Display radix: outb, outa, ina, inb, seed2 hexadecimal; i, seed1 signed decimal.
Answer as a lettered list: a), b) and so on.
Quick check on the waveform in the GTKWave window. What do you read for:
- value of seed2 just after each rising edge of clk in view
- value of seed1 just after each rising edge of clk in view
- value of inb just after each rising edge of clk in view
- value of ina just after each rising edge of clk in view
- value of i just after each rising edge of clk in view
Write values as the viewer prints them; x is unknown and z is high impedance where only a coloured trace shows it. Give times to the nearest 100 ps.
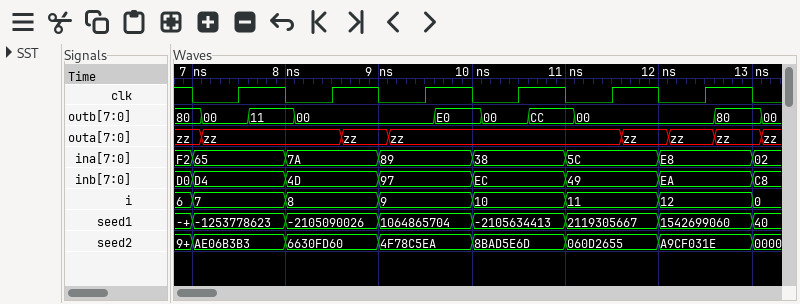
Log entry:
a) AE06B3B3, 6630FD60, 4F78C5EA, 8BAD5E6D, 060D2655, A9CF031E
b) -1253778623, -2105090026, 1064865704, -2105634413, 2119305667, 1542699060
c) D4, 4D, 97, EC, 49, EA
d) 65, 7A, 89, 38, 5C, E8
e) 7, 8, 9, 10, 11, 12
